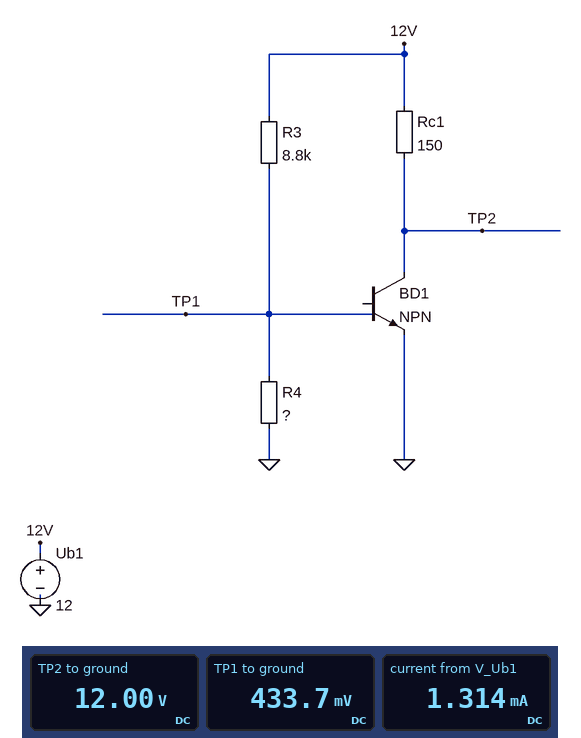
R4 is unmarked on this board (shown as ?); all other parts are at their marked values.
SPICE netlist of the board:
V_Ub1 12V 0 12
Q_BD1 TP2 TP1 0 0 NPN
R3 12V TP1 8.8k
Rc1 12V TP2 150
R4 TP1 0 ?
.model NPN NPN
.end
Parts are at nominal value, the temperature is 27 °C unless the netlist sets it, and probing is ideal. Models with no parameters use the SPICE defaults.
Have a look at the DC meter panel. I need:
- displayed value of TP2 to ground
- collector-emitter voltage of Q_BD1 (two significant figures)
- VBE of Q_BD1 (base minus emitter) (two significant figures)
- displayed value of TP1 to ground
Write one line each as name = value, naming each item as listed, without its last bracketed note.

displayed value of TP2 to ground = 12.00 V
collector-emitter voltage of Q_BD1 = 12 V
VBE of Q_BD1 (base minus emitter) = 430 mV
displayed value of TP1 to ground = 433.7 mV
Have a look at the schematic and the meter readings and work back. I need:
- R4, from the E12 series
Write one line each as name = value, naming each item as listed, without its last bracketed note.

R4, from the E12 series = 330 Ω
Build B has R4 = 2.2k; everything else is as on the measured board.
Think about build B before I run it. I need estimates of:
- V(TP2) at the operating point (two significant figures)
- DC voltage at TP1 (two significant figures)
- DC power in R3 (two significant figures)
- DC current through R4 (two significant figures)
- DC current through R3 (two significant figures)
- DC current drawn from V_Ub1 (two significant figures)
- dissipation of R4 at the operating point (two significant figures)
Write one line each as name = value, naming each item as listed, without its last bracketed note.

V(TP2) at the operating point = 180 mV
DC voltage at TP1 = 890 mV
DC power in R3 = 14 mW
DC current through R4 = 400 µA
DC current through R3 = 1.3 mA
DC current drawn from V_Ub1 = 80 mA
dissipation of R4 at the operating point = 360 µW
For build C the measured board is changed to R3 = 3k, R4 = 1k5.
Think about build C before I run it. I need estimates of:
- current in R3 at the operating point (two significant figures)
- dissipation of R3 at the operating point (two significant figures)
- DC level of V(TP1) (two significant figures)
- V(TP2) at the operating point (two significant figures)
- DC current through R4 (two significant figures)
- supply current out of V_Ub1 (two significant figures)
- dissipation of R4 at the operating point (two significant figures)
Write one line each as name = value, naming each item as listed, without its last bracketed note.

current in R3 at the operating point = 3.7 mA
dissipation of R3 at the operating point = 41 mW
DC level of V(TP1) = 890 mV
V(TP2) at the operating point = 93 mV
DC current through R4 = 590 µA
supply current out of V_Ub1 = 83 mA
dissipation of R4 at the operating point = 530 µW
